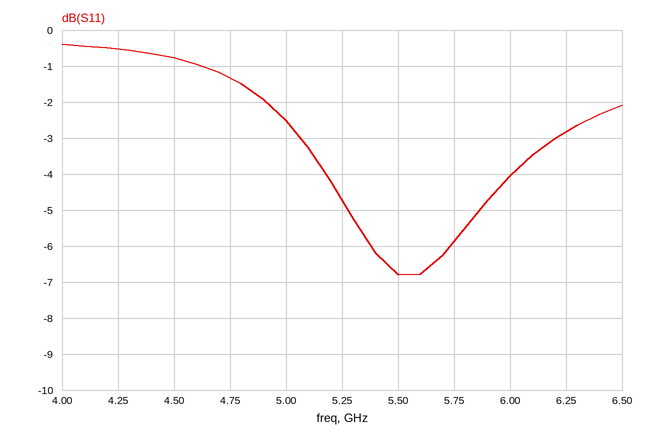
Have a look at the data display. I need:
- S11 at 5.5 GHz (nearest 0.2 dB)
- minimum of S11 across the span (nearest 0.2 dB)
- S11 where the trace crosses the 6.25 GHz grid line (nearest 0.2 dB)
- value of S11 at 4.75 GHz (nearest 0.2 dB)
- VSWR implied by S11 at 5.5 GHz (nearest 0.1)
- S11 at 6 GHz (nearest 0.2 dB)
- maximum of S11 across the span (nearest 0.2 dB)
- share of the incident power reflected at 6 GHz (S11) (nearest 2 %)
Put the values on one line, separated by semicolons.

-6.8 dB; -6.8 dB; -2.8 dB; -1.4 dB; 2.7; -4.0 dB; -0.4 dB; 40 %
